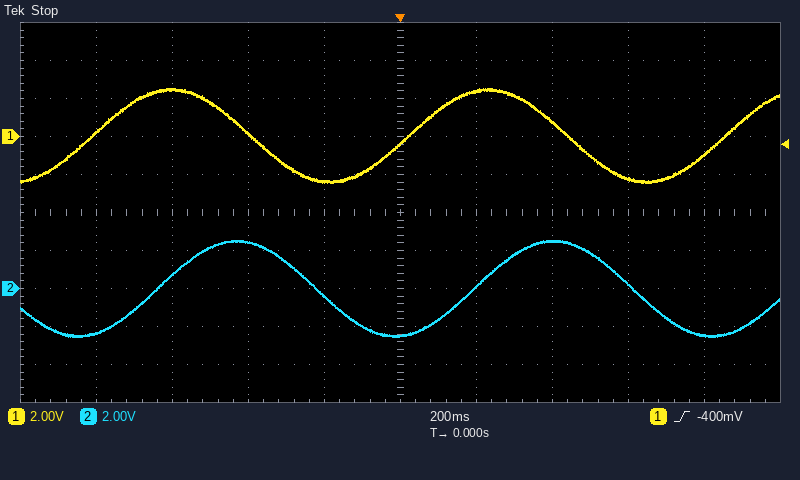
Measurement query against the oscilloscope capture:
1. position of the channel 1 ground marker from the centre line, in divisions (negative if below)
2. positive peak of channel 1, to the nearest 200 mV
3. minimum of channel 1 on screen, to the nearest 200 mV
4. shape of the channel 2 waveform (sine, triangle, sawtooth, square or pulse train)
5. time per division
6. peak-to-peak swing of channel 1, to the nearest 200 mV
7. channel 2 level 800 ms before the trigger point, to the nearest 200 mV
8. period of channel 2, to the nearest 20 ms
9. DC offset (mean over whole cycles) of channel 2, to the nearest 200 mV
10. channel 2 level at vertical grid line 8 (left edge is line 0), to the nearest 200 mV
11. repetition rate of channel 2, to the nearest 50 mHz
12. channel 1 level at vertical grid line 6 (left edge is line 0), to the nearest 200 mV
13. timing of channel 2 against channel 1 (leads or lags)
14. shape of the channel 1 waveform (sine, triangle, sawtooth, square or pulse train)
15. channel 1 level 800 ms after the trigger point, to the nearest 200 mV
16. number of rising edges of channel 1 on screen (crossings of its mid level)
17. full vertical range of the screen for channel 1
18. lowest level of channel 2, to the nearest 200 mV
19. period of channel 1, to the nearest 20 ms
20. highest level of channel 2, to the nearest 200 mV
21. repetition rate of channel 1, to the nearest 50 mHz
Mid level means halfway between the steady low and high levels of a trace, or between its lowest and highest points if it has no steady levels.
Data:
+2.0 div
2.6 V
-2.4 V
sine
200 ms
5.0 V
-2.4 V
840 ms
0.0 V
200 mV
1.20 Hz
2.4 V
lags
sine
-1.0 V
3
20 V
-2.6 V
840 ms
2.6 V
1.20 Hz
